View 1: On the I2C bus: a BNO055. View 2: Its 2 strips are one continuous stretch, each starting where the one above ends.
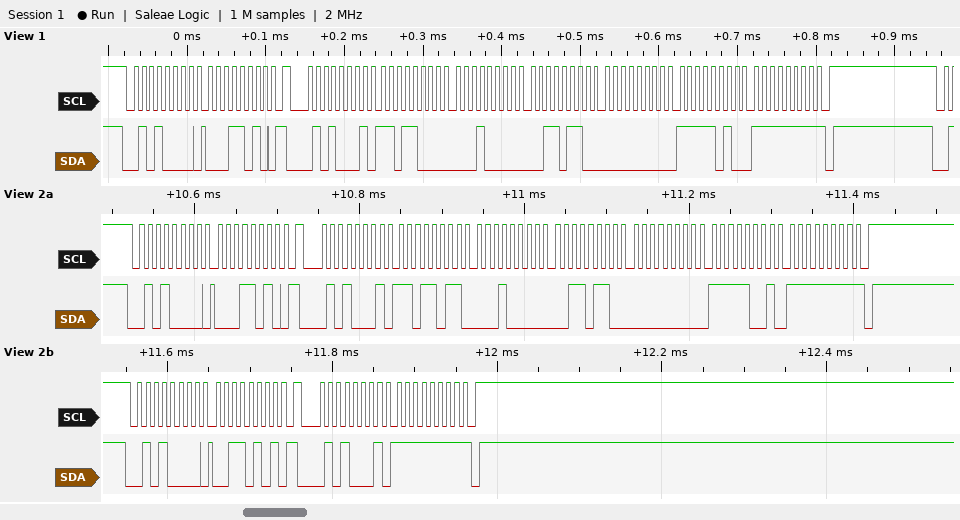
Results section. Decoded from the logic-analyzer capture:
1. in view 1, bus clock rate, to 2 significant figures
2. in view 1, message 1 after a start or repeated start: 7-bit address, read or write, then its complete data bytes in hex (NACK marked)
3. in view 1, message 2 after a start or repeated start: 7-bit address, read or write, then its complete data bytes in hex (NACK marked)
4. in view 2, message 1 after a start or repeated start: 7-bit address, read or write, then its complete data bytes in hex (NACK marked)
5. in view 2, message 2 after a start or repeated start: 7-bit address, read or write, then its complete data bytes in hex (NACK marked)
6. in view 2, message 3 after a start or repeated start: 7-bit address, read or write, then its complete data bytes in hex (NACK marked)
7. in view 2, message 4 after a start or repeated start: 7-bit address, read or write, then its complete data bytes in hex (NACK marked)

100 kHz
0x28 write: 1A
0x28 read: D8 10 36 00 FA FF NACK
0x28 write: 1A
0x28 read: DB 10 36 00 F9 FF NACK
0x28 write: 35
0x28 read: FF NACK
